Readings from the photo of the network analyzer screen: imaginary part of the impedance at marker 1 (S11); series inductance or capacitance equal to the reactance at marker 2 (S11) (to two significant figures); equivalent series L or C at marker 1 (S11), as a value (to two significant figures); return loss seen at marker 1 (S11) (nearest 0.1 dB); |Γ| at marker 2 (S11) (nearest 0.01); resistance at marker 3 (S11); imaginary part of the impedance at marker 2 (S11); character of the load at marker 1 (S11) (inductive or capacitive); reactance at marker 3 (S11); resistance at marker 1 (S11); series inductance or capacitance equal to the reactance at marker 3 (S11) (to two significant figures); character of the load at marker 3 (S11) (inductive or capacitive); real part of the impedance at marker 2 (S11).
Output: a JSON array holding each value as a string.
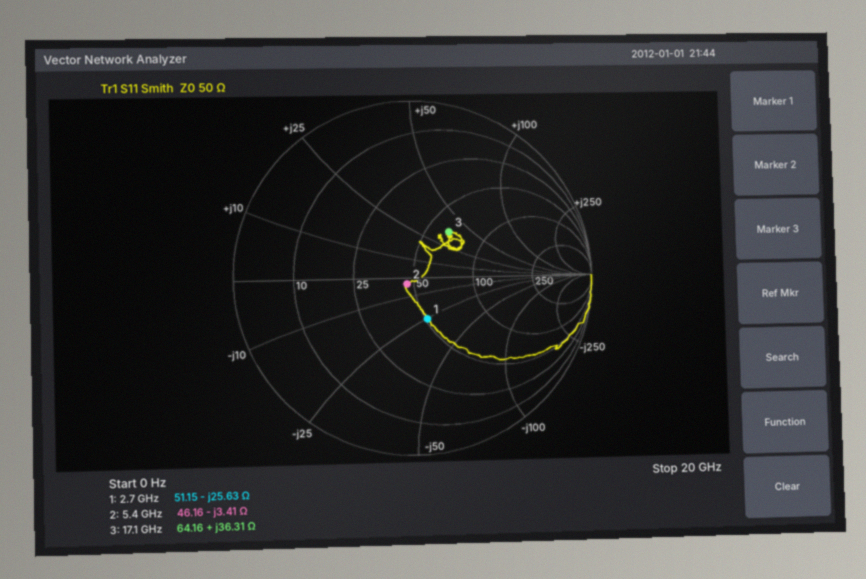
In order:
["-25.63 Ω", "8.6 pF", "2.3 pF", "12.2 dB", "0.05", "64.16 Ω", "-3.41 Ω", "capacitive", "+36.31 Ω", "51.15 Ω", "340 pH", "inductive", "46.16 Ω"]
